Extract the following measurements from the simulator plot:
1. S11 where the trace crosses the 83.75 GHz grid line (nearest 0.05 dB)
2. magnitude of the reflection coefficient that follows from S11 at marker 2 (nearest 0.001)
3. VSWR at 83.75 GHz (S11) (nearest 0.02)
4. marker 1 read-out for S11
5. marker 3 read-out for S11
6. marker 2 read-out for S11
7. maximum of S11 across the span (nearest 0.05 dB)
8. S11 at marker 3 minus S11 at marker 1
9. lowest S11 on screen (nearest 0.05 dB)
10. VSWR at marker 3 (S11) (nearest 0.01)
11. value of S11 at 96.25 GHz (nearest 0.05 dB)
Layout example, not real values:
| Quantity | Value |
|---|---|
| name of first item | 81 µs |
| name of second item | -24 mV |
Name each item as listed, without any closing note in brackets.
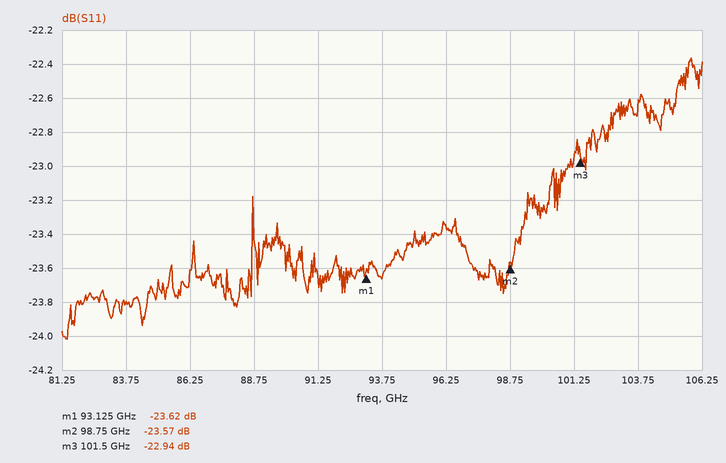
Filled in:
| Quantity | Value |
|---|---|
| S11 where the trace crosses the 83.75 GHz grid line | -23.80 dB |
| magnitude of the reflection coefficient that follows from S11 at marker 2 | 0.066 |
| VSWR at 83.75 GHz (S11) | 1.14 |
| marker 1 read-out for S11 | -23.62 dB |
| marker 3 read-out for S11 | -22.94 dB |
| marker 2 read-out for S11 | -23.57 dB |
| maximum of S11 across the span | -22.35 dB |
| S11 at marker 3 minus S11 at marker 1 | 0.68 dB |
| lowest S11 on screen | -24.00 dB |
| VSWR at marker 3 (S11) | 1.15 |
| value of S11 at 96.25 GHz | -23.35 dB |
